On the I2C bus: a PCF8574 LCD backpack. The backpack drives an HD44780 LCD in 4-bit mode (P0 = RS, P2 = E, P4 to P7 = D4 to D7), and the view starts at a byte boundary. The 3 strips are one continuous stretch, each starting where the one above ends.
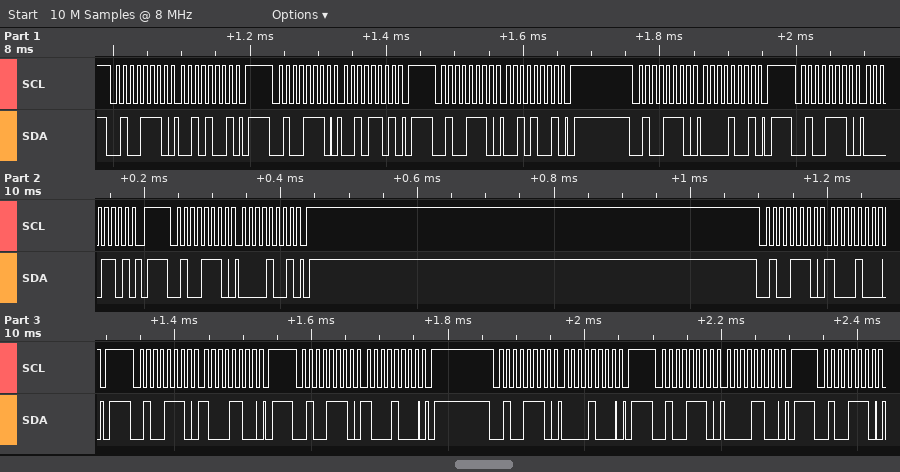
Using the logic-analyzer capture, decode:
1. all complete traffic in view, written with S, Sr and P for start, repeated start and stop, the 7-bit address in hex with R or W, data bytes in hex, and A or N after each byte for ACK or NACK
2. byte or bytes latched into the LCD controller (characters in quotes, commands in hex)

S 27W A 29 A P S 27W A 2D A P S 27W A 29 A P S 27W A 09 A P S 27W A 0D A P S 27W A 09 A P S 27W A 88 A P S 27W A 8C A P S 27W A 88 A P S 27W A 08 A P S 27W A 0C A P S 27W A
' '
